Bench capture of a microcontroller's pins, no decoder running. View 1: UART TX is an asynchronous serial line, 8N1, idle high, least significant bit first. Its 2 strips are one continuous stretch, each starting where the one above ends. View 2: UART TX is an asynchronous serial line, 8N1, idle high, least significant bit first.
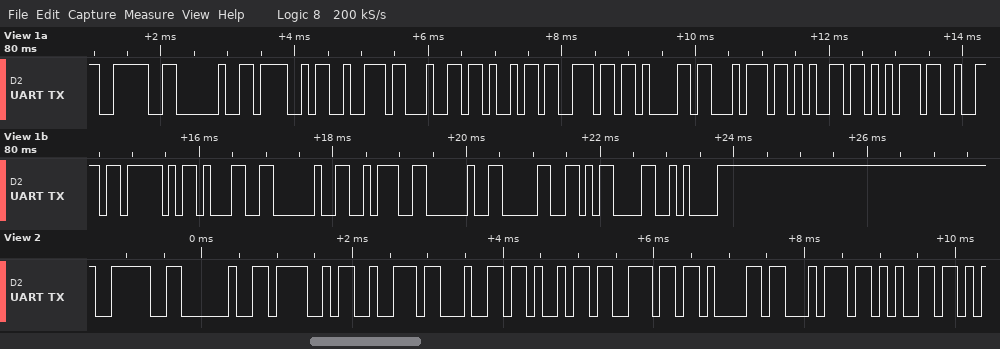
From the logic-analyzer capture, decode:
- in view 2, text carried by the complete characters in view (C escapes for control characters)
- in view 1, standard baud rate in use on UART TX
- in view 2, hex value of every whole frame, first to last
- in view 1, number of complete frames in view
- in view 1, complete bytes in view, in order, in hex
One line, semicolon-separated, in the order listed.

"> Ordinate"; 9600 baud; 3E 20 4F 72 64 69 6E 61 74 65; 20; 3E 20 4F 72 64 69 6E 61 74 65 75 72 5F 31 20 3A 20 30 0D 0A
